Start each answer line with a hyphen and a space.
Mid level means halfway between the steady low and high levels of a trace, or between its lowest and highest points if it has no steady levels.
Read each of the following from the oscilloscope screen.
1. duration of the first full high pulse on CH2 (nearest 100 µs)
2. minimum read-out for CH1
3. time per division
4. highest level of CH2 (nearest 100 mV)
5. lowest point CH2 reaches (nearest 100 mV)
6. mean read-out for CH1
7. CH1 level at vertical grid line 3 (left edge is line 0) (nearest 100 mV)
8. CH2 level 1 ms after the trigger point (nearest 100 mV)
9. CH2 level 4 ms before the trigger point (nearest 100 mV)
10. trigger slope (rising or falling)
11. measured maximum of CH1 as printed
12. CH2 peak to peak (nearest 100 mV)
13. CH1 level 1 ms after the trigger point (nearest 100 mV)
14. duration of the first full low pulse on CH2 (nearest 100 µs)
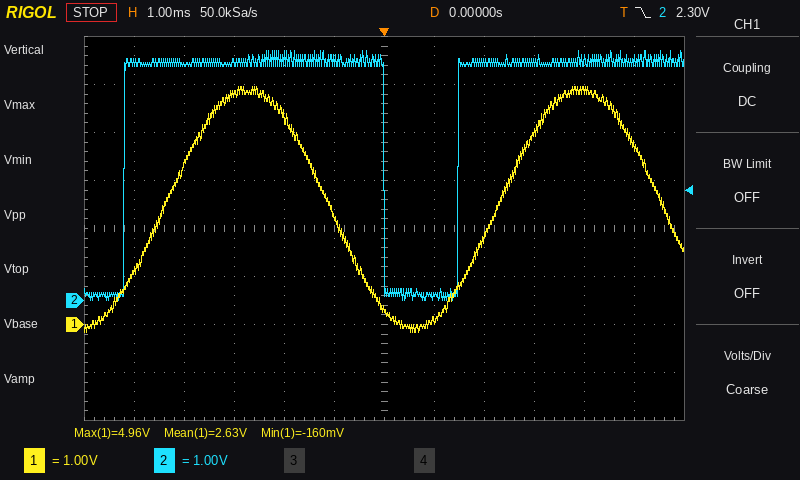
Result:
- 5.2 ms
- -160 mV
- 1 ms
- 5.2 V
- 0.0 V
- 2.63 V
- 4.8 V
- 100 mV
- 4.9 V
- falling
- 4.96 V
- 5.2 V
- 100 mV
- 1.5 ms
